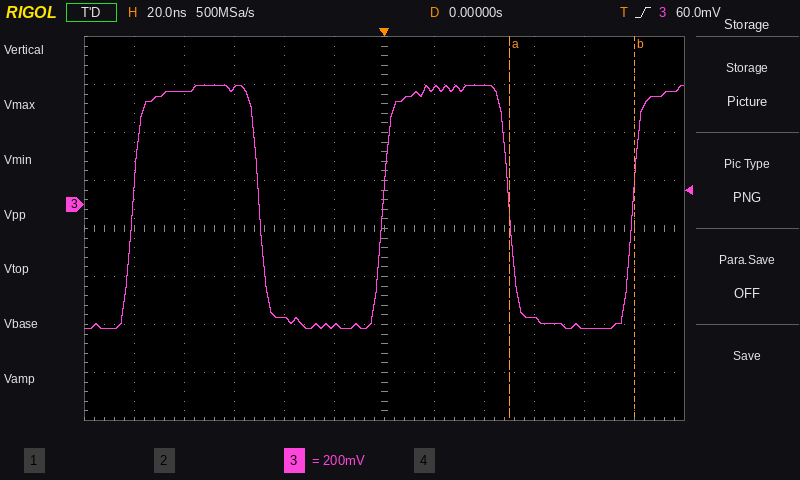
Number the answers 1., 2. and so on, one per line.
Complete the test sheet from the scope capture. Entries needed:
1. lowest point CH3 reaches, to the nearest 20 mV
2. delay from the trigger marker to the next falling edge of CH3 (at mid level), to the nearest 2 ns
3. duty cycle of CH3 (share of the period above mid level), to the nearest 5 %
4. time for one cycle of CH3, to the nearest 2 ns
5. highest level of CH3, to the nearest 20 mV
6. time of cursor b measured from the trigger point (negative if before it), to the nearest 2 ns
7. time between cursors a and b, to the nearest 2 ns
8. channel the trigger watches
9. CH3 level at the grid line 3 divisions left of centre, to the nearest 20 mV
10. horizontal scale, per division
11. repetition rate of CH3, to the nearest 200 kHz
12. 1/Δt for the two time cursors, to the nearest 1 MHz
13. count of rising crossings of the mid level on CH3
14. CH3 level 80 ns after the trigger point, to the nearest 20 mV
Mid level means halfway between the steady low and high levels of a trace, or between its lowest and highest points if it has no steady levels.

1. -520 mV
2. 50 ns
3. 50 %
4. 100 ns
5. 500 mV
6. +100 ns
7. 50 ns
8. CH3
9. 480 mV
10. 20 ns
11. 10.0 MHz
12. 20 MHz
13. 3
14. -520 mV
